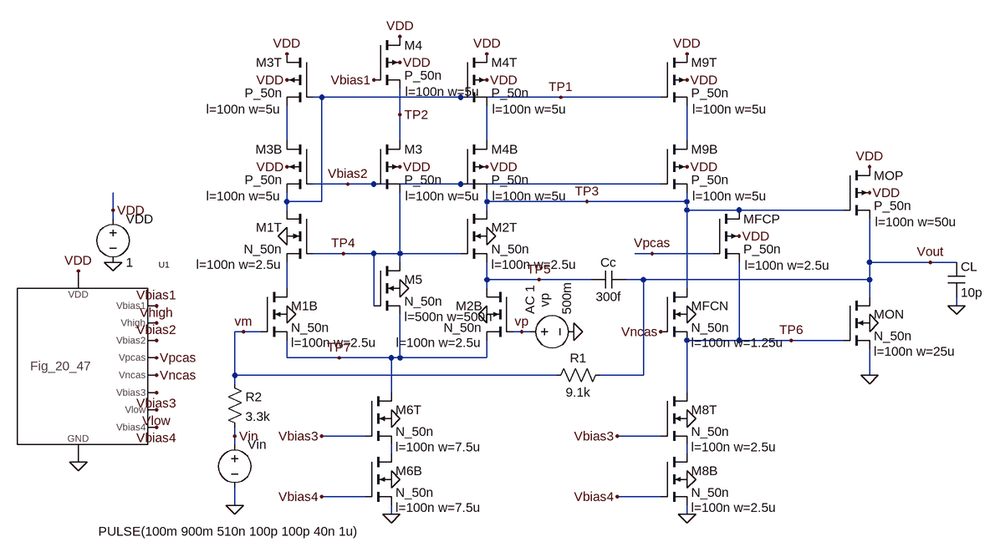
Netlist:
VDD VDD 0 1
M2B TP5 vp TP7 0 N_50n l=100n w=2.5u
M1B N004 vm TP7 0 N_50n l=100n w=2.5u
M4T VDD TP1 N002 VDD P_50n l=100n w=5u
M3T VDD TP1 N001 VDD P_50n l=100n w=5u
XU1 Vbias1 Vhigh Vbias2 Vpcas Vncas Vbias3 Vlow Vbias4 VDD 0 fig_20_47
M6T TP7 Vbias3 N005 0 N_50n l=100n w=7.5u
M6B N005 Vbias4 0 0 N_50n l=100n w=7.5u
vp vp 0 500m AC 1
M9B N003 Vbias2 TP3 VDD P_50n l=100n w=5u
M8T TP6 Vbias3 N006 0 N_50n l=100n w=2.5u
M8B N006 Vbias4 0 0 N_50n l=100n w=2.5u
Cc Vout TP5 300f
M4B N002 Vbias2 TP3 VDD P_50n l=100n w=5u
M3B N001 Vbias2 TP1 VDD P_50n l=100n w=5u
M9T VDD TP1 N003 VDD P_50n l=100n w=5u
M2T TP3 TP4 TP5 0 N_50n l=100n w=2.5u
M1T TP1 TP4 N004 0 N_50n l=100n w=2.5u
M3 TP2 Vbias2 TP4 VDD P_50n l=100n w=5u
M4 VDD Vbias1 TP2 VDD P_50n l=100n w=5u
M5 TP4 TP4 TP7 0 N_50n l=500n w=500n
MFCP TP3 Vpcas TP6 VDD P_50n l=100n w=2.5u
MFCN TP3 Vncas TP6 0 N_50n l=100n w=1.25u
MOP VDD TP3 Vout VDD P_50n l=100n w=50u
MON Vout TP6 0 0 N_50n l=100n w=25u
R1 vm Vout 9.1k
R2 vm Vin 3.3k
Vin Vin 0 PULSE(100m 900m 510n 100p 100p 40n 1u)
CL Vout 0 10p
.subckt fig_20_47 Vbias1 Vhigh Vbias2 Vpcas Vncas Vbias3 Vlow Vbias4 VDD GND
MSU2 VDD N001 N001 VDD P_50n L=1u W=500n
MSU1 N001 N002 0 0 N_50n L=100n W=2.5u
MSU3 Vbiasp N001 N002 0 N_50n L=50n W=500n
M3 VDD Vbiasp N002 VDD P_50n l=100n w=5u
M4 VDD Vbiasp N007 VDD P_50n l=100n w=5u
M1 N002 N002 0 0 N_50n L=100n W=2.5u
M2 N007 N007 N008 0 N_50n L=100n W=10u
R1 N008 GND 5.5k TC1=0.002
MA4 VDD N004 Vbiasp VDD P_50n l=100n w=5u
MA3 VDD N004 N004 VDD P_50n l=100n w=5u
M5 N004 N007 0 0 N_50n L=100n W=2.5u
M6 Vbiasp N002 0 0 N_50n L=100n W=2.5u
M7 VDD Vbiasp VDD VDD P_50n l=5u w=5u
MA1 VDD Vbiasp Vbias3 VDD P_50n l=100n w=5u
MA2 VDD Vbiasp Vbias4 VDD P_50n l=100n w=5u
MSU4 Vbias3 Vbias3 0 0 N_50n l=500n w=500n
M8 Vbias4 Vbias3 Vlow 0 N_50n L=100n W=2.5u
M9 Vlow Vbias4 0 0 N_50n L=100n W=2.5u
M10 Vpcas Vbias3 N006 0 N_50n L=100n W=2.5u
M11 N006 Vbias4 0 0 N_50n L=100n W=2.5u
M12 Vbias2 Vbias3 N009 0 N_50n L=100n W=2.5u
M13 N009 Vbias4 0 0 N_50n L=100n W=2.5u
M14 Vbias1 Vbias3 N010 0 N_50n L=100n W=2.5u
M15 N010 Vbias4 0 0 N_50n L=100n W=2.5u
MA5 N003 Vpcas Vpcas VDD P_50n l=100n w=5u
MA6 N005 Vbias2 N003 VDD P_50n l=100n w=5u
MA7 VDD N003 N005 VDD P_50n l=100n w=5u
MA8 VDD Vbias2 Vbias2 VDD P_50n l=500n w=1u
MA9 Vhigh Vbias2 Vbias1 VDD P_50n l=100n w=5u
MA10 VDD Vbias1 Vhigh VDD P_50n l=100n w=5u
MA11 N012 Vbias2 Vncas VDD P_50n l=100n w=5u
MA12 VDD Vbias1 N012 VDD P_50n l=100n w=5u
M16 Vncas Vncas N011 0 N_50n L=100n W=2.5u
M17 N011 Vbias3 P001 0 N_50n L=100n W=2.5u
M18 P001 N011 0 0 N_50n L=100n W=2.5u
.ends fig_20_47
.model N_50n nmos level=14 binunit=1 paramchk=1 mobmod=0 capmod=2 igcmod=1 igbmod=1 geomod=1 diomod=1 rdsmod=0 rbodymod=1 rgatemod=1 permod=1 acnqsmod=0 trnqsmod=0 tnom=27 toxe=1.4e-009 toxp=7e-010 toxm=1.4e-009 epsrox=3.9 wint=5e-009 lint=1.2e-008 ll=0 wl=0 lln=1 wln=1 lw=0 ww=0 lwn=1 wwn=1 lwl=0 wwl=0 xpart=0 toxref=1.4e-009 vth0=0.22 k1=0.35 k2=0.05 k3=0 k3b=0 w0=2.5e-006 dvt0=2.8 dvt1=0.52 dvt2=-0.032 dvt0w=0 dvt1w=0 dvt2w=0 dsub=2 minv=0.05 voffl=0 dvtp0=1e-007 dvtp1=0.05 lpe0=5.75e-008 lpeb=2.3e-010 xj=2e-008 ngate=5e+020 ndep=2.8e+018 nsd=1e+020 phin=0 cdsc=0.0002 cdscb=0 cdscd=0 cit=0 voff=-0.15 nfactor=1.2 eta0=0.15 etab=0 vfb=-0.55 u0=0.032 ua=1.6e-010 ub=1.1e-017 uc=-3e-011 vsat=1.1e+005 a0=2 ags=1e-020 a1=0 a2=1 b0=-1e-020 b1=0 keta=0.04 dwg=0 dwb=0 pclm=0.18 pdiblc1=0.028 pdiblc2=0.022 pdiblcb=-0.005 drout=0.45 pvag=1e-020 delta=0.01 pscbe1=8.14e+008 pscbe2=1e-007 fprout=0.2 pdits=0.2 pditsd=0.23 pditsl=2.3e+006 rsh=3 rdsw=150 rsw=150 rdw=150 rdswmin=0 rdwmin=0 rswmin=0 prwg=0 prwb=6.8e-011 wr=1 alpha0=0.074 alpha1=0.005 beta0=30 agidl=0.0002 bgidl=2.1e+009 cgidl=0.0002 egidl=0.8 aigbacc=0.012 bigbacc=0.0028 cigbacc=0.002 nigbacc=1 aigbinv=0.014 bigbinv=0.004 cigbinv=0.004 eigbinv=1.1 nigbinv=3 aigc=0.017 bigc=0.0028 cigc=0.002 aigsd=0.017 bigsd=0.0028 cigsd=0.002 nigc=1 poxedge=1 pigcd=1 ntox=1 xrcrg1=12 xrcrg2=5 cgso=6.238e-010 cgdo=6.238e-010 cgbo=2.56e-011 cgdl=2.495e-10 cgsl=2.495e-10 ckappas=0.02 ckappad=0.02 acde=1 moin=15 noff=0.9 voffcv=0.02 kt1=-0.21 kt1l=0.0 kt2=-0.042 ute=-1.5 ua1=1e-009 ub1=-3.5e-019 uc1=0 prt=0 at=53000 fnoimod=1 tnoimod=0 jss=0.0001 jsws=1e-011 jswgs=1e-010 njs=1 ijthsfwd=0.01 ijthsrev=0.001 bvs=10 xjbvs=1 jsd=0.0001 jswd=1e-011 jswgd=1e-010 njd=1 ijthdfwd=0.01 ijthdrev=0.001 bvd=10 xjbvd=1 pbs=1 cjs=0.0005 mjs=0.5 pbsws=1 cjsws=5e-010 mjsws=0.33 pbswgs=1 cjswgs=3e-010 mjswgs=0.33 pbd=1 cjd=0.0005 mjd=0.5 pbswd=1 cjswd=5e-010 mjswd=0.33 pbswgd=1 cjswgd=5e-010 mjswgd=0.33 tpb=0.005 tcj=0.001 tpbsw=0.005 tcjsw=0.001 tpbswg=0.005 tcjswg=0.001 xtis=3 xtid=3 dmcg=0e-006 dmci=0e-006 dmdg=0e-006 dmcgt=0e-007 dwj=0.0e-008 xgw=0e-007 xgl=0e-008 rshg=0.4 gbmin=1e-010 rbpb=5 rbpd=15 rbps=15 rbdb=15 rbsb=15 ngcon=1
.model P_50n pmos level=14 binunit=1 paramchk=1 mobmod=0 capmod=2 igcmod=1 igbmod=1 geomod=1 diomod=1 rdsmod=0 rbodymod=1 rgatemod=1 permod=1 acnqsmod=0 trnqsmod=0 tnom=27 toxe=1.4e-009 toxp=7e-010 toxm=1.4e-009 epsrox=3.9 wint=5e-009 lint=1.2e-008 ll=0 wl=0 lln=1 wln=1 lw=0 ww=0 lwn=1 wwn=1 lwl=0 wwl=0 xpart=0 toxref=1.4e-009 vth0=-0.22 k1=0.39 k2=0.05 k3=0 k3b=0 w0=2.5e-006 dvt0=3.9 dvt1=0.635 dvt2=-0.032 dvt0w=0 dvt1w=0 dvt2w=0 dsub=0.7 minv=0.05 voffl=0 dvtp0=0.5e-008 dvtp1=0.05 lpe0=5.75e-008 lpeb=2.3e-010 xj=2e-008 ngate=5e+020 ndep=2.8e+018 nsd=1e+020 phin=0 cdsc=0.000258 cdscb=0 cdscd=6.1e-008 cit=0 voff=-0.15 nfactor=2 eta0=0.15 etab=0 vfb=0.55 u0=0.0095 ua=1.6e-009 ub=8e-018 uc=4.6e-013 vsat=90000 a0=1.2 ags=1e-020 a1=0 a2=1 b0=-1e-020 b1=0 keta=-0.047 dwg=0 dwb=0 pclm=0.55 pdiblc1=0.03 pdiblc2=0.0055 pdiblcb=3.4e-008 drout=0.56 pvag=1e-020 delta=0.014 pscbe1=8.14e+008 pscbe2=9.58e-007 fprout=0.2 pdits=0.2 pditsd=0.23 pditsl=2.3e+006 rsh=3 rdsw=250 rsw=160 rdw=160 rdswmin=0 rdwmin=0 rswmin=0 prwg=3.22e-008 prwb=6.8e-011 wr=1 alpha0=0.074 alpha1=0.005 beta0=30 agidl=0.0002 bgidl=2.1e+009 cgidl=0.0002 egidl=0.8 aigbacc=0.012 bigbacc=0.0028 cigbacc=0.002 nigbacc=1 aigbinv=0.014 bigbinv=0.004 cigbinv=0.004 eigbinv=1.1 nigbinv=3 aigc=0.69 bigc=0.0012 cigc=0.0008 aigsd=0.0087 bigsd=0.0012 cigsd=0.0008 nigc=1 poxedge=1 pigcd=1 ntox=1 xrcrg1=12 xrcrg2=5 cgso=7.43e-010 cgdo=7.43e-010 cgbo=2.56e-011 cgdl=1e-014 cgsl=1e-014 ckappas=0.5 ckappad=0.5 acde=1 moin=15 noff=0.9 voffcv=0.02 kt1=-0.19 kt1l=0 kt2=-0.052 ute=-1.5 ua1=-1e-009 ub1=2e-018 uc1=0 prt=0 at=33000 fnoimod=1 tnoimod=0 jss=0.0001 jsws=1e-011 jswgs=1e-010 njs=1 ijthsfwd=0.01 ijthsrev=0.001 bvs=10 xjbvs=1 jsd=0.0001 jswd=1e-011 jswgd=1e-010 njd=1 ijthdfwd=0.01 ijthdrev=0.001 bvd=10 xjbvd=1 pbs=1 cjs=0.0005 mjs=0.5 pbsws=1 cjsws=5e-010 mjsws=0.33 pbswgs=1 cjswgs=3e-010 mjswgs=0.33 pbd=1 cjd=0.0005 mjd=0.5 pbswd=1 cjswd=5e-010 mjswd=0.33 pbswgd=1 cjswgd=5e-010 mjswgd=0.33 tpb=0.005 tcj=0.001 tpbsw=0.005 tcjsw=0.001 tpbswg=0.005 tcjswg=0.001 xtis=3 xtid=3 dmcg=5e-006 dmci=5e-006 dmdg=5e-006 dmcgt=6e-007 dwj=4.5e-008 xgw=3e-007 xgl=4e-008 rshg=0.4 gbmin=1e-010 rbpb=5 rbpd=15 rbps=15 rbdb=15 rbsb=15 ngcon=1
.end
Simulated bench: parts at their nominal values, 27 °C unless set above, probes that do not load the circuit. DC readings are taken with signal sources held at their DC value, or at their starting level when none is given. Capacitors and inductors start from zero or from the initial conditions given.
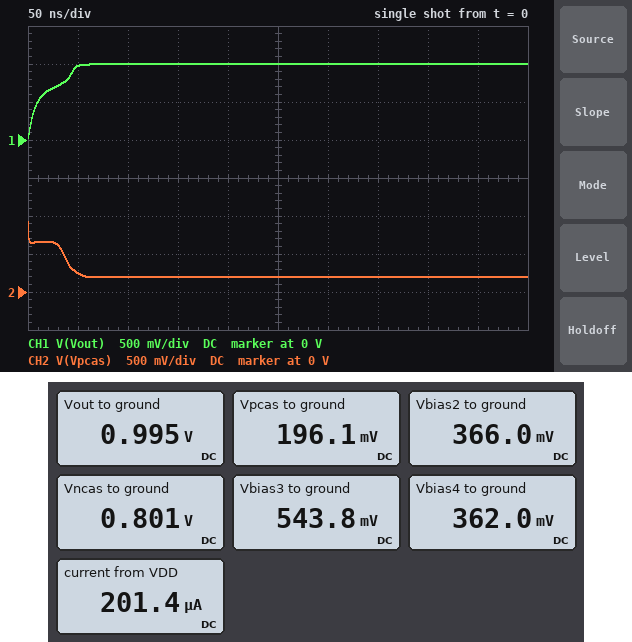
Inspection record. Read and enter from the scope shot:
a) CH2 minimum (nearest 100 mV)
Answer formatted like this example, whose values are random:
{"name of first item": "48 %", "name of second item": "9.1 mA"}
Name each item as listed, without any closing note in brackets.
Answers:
{"CH2 minimum": "200 mV"}
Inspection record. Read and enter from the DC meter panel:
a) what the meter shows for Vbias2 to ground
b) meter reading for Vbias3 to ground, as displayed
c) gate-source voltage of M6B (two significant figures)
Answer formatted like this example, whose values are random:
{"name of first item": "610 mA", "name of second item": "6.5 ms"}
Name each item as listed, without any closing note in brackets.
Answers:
{"what the meter shows for Vbias2 to ground": "366.0 mV", "meter reading for Vbias3 to ground, as displayed": "543.8 mV", "gate-source voltage of M6B": "360 mV"}
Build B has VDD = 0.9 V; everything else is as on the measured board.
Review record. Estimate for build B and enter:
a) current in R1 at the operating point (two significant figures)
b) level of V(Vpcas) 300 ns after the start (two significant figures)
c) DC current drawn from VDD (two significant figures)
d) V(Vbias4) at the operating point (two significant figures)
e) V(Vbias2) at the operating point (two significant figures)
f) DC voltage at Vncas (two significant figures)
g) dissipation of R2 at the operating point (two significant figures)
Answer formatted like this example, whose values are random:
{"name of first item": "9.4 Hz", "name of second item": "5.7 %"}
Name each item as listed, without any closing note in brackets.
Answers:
{"current in R1 at the operating point": "64 µA", "level of V(Vpcas) 300 ns after the start": "110 mV", "DC current drawn from VDD": "190 µA", "V(Vbias4) at the operating point": "360 mV", "V(Vbias2) at the operating point": "270 mV", "DC voltage at Vncas": "790 mV", "dissipation of R2 at the operating point": "14 µW"}
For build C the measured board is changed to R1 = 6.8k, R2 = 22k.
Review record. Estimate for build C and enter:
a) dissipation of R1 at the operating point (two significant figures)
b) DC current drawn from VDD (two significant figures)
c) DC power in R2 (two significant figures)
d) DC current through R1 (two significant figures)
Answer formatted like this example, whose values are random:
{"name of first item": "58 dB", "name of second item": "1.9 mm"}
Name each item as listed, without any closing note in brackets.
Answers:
{"dissipation of R1 at the operating point": "2.3 µW", "DC current drawn from VDD": "270 µA", "DC power in R2": "7.4 µW", "DC current through R1": "18 µA"}
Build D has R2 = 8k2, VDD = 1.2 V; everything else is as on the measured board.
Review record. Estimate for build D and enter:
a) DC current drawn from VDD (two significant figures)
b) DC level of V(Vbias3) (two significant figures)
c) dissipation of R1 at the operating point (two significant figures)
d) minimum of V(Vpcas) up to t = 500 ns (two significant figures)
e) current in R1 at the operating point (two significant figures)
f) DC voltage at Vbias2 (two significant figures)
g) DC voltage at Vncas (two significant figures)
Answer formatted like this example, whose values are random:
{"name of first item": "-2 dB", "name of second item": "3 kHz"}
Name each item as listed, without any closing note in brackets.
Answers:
{"DC current drawn from VDD": "320 µA", "DC level of V(Vbias3)": "550 mV", "dissipation of R1 at the operating point": "22 µW", "minimum of V(Vpcas) up to t = 500 ns": "390 mV", "current in R1 at the operating point": "49 µA", "DC voltage at Vbias2": "560 mV", "DC voltage at Vncas": "810 mV"}
